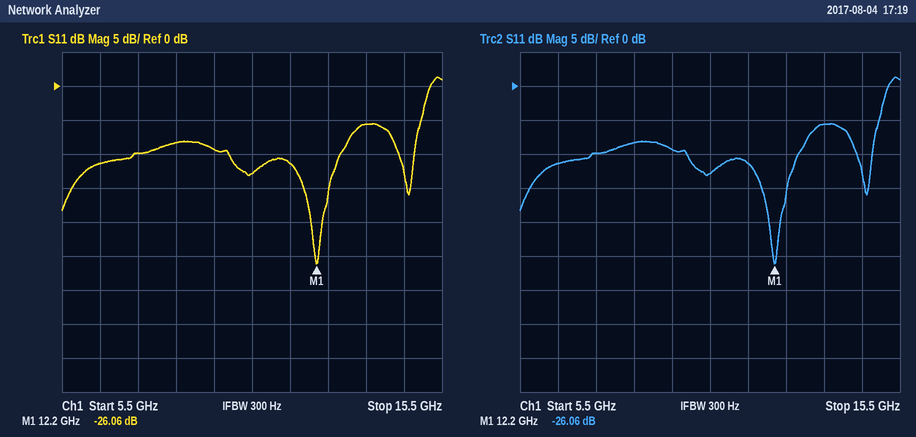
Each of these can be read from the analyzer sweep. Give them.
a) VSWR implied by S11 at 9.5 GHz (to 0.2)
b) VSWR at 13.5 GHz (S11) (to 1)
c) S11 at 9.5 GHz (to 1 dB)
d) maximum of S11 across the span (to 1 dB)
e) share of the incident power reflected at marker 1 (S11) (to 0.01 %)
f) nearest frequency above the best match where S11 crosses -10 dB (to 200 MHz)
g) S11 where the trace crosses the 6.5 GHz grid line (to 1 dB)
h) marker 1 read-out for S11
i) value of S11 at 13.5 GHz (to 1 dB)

2.0
3
-9 dB
1 dB
0.25 %
12.8 GHz
-11 dB
-26.06 dB
-6 dB
